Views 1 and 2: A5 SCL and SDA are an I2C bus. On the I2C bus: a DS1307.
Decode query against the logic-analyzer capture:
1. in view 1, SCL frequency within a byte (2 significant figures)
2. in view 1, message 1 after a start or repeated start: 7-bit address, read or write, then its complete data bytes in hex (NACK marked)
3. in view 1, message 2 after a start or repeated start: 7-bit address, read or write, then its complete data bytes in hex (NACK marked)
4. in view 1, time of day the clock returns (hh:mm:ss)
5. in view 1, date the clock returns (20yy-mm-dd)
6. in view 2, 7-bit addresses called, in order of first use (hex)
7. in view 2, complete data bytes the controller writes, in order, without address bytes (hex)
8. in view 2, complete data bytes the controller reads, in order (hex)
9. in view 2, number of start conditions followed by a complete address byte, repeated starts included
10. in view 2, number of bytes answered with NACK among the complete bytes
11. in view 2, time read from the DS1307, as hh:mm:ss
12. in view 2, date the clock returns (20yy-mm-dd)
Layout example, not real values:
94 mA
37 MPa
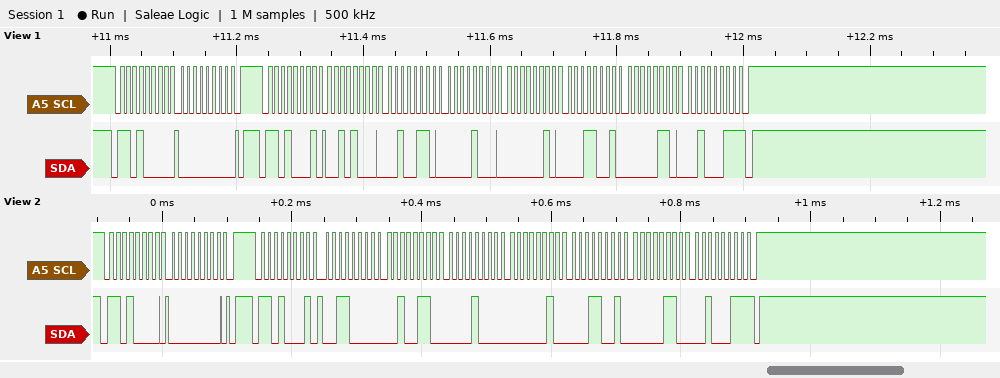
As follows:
100 kHz
0x68 write: 00
0x68 read: 28 26 08 02 19 06 23 NACK
08:26:28
2023-06-19
0x68
00
30 26 08 02 19 06 23
2
1
08:26:30
2023-06-19
